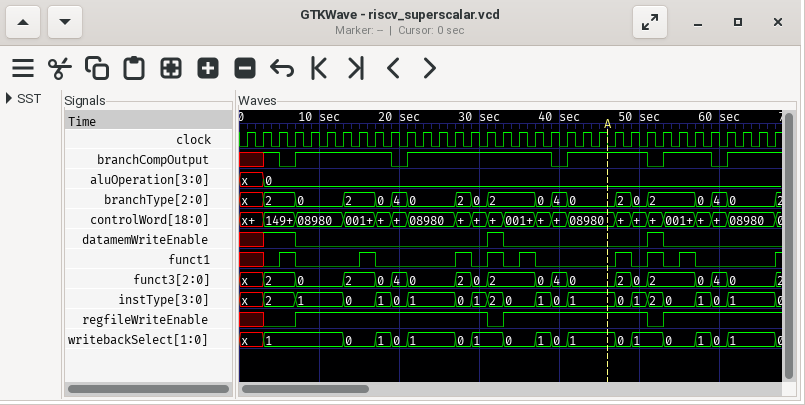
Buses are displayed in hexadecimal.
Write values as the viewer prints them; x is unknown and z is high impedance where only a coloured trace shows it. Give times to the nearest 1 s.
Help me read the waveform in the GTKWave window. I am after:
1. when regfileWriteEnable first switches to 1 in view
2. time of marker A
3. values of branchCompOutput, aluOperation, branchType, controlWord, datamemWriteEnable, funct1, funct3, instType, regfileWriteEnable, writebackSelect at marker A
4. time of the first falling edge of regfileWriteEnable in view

7 s
46 s
branchCompOutput=1, aluOperation=0, branchType=0, controlWord=08980, datamemWriteEnable=0, funct1=0, funct3=0, instType=1, regfileWriteEnable=1, writebackSelect=1
31 s
